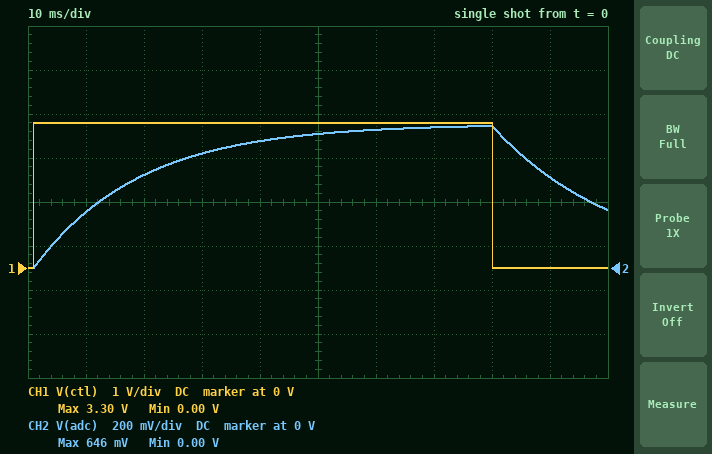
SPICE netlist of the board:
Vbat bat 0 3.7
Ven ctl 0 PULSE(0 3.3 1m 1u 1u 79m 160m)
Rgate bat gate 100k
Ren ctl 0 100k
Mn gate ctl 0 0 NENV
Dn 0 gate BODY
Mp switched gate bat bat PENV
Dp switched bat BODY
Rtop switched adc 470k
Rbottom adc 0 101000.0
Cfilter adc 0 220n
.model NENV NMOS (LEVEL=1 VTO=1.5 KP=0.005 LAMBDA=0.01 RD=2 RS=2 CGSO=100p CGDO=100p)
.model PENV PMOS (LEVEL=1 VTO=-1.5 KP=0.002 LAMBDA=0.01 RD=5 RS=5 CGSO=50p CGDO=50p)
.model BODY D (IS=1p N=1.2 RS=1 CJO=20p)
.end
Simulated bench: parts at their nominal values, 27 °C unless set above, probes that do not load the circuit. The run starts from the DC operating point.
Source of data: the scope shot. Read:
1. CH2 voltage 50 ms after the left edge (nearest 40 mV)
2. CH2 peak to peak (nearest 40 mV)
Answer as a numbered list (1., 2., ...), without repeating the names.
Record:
1. 600 mV
2. 640 mV
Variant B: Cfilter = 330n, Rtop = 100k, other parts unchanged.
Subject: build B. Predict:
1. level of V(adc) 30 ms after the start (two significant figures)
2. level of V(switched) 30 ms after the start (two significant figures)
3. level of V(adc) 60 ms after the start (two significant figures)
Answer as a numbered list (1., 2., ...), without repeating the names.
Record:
1. 1.5 V
2. 3.7 V
3. 1.8 V
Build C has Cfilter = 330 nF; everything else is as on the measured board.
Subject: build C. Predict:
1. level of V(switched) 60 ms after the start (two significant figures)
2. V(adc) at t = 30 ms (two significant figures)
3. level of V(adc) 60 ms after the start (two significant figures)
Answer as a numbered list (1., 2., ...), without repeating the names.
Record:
1. 3.7 V
2. 430 mV
3. 580 mV
